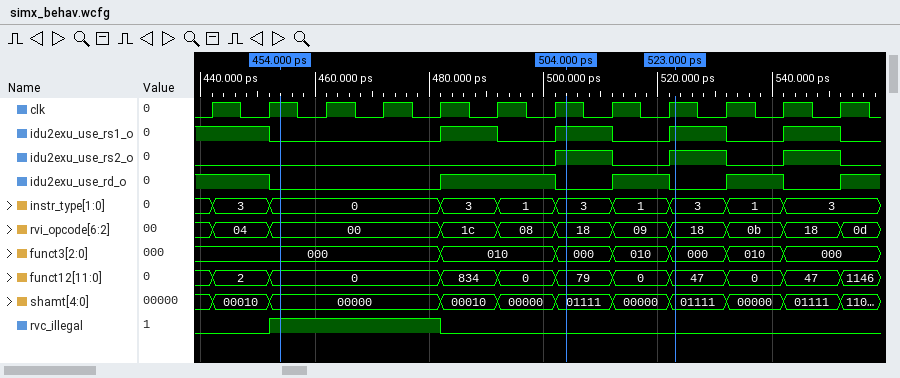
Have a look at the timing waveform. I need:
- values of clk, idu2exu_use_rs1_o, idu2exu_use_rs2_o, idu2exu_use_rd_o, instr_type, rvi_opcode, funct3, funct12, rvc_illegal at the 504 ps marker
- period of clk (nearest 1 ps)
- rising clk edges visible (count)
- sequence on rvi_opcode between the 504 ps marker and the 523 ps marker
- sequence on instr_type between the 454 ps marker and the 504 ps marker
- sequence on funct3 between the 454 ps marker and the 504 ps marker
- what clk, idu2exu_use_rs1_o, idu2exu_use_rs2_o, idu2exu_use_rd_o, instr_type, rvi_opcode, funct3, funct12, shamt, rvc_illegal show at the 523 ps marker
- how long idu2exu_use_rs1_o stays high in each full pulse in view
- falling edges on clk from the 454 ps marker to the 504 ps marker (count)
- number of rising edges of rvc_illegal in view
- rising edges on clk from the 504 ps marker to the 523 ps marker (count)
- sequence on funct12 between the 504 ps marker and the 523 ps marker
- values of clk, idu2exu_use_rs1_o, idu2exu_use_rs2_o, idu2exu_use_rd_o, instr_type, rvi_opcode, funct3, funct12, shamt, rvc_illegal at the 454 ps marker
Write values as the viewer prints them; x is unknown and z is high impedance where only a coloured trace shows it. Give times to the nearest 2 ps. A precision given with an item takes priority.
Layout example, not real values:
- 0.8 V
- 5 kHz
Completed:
- clk=1, idu2exu_use_rs1_o=1, idu2exu_use_rs2_o=1, idu2exu_use_rd_o=0, instr_type=3, rvi_opcode=18, funct3=000, funct12=79, rvc_illegal=0
- 10 ps
- 12
- 18, 09, 18
- 0, 3, 1, 3
- 000, 010, 000
- clk=1, idu2exu_use_rs1_o=1, idu2exu_use_rs2_o=1, idu2exu_use_rd_o=0, instr_type=3, rvi_opcode=18, funct3=000, funct12=47, shamt=01111, rvc_illegal=0
- 10 ps, 10 ps, 10 ps, 10 ps
- 5
- 1
- 2
- 79, 0, 47
- clk=1, idu2exu_use_rs1_o=0, idu2exu_use_rs2_o=0, idu2exu_use_rd_o=0, instr_type=0, rvi_opcode=00, funct3=000, funct12=0, shamt=00000, rvc_illegal=1
